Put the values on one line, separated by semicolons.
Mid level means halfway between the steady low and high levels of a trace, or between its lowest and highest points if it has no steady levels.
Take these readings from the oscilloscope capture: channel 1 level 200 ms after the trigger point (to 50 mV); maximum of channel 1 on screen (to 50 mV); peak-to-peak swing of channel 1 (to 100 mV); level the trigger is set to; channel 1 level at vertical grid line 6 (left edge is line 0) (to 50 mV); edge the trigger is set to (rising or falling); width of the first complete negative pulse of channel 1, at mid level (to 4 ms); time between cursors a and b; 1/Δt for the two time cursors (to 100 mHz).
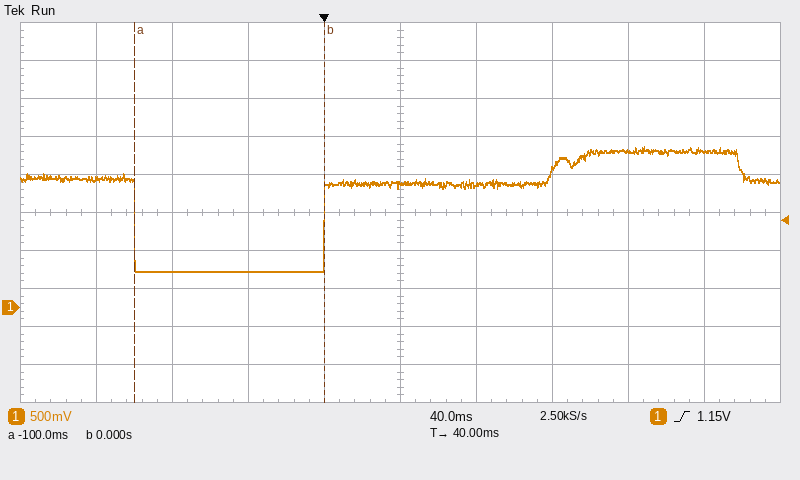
2.05 V; 2.10 V; 1.60 V; 1.15 V; 1.60 V; rising; 100 ms; 100 ms; 10.0 Hz
